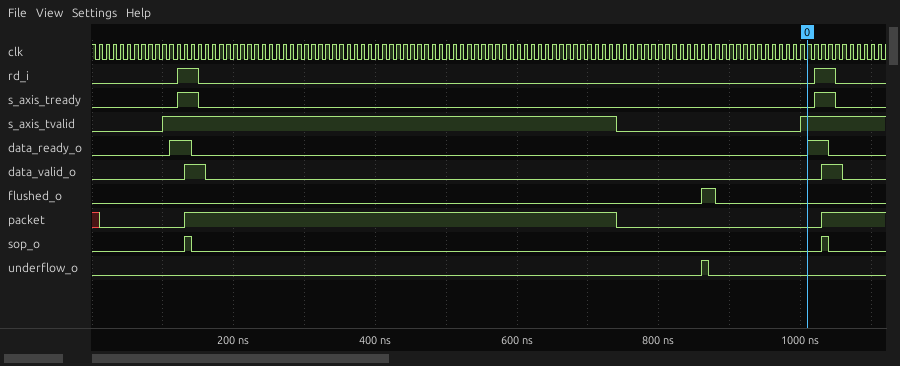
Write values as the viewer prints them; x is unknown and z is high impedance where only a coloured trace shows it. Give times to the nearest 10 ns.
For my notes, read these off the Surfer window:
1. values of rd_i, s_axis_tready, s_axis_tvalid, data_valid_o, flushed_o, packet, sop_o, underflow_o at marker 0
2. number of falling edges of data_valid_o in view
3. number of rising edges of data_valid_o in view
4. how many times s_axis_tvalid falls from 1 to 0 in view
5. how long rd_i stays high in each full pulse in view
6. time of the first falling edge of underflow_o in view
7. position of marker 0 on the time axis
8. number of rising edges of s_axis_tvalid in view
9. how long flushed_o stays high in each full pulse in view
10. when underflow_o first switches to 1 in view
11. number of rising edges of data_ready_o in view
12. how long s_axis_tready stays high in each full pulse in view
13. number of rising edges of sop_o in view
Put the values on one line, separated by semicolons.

rd_i=0, s_axis_tready=0, s_axis_tvalid=1, data_valid_o=0, flushed_o=0, packet=0, sop_o=0, underflow_o=0; 2; 2; 1; 30 ns, 30 ns; 870 ns; 1010 ns; 2; 20 ns; 860 ns; 2; 30 ns, 30 ns; 2
